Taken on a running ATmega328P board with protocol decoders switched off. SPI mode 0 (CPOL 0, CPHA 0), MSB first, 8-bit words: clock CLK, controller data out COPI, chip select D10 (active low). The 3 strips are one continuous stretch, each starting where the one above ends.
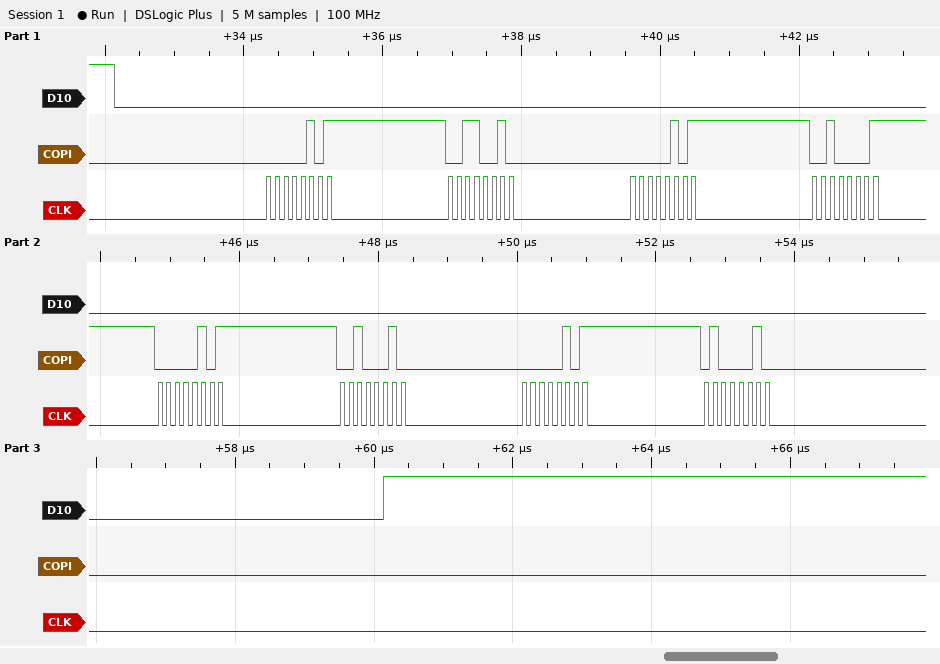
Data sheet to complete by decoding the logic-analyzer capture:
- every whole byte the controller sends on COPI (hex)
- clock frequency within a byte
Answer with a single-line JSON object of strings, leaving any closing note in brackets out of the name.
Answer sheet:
{"every whole byte the controller sends on COPI": "05 32 05 21 05 22 05 42", "clock frequency within a byte": "8 MHz"}
